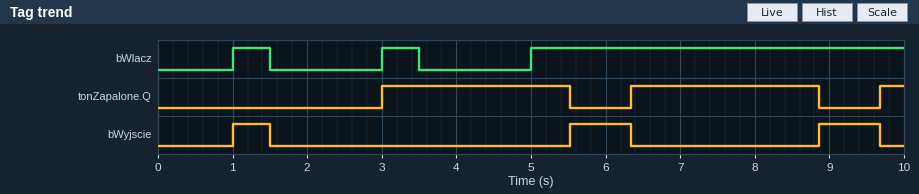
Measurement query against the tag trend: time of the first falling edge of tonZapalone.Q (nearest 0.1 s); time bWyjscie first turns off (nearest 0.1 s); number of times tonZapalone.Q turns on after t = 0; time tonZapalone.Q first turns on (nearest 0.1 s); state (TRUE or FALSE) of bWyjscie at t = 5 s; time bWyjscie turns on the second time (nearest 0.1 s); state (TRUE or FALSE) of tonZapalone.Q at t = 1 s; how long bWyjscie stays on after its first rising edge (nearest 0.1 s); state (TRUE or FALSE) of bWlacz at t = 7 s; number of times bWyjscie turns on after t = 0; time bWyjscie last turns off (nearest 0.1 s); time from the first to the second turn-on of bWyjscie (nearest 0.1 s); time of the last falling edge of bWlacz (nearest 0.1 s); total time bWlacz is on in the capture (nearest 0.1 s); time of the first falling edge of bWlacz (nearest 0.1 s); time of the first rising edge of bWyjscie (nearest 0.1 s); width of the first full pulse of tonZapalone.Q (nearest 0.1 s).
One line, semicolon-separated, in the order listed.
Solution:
5.5 s; 1.5 s; 3; 3.0 s; FALSE; 5.5 s; FALSE; 0.5 s; TRUE; 3; 9.7 s; 4.5 s; 3.5 s; 6.0 s; 1.5 s; 1.0 s; 2.5 s
